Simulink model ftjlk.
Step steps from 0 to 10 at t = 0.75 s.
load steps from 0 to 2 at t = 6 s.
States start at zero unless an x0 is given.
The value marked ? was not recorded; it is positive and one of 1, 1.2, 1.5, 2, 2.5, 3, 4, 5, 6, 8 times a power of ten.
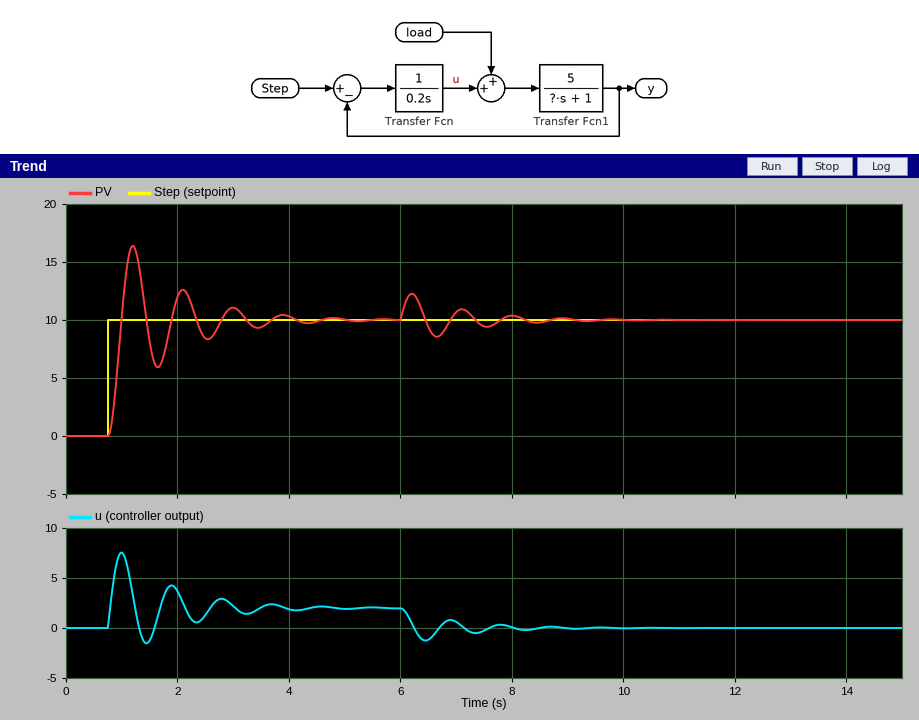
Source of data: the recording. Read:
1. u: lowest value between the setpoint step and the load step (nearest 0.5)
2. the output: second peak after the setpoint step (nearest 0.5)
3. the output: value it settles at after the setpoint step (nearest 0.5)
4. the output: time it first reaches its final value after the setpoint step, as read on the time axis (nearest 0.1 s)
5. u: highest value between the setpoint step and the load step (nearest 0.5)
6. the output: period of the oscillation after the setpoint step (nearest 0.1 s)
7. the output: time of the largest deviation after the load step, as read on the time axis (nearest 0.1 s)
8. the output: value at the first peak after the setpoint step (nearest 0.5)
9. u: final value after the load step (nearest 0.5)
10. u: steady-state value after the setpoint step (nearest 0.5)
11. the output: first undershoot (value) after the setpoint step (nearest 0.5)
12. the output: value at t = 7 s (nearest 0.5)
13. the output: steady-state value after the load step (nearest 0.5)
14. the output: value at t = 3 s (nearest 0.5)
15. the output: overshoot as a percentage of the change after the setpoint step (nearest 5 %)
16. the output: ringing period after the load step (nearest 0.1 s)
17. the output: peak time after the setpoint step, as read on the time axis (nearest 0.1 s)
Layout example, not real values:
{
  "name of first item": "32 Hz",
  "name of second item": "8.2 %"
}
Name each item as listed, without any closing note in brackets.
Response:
{
  "u: lowest value between the setpoint step and the load step": "-1.5",
  "the output: second peak after the setpoint step": "12.5",
  "the output: value it settles at after the setpoint step": "10.0",
  "the output: time it first reaches its final value after the setpoint step, as read on the time axis": "1.0 s",
  "u: highest value between the setpoint step and the load step": "7.5",
  "the output: period of the oscillation after the setpoint step": "0.9 s",
  "the output: time of the largest deviation after the load step, as read on the time axis": "6.2 s",
  "the output: value at the first peak after the setpoint step": "16.5",
  "u: final value after the load step": "0.0",
  "u: steady-state value after the setpoint step": "2.0",
  "the output: first undershoot (value) after the setpoint step": "6.0",
  "the output: value at t = 7 s": "10.5",
  "the output: steady-state value after the load step": "10.0",
  "the output: value at t = 3 s": "11.0",
  "the output: overshoot as a percentage of the change after the setpoint step": "65 %",
  "the output: ringing period after the load step": "0.9 s",
  "the output: peak time after the setpoint step, as read on the time axis": "1.2 s"
}
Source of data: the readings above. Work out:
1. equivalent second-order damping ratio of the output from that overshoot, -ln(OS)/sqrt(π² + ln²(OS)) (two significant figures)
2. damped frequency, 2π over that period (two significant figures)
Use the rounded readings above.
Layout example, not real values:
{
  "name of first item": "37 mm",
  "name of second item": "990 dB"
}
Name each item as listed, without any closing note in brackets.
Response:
{
  "equivalent second-order damping ratio of the output from that overshoot, -ln(OS)/sqrt(π² + ln²(OS))": "0.14",
  "damped frequency, 2π over that period": "7.0 rad/s"
}
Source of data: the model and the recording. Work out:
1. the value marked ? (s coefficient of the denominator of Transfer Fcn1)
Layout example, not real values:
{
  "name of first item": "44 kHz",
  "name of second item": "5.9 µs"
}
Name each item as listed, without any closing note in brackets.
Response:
{
  "the value marked ?": "0.5"
}
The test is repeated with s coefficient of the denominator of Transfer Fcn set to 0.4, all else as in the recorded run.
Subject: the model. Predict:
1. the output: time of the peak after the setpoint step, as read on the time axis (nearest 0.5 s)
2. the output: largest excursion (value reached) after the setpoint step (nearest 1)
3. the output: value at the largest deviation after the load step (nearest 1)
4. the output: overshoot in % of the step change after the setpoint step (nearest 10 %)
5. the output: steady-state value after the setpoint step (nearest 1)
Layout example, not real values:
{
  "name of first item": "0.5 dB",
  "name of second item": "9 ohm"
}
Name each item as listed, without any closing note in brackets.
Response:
{
  "the output: time of the peak after the setpoint step, as read on the time axis": "1.5 s",
  "the output: largest excursion (value reached) after the setpoint step": "15",
  "the output: value at the largest deviation after the load step": "13",
  "the output: overshoot in % of the step change after the setpoint step": "50 %",
  "the output: steady-state value after the setpoint step": "10"
}
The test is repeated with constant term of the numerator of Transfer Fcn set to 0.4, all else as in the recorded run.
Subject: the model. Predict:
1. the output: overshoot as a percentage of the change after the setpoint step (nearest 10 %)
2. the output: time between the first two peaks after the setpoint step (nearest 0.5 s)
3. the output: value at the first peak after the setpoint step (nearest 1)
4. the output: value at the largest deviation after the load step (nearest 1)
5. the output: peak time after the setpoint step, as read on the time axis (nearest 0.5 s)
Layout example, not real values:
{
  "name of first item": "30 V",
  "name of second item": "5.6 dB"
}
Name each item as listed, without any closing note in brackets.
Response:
{
  "the output: overshoot as a percentage of the change after the setpoint step": "50 %",
  "the output: time between the first two peaks after the setpoint step": "1.5 s",
  "the output: value at the first peak after the setpoint step": "15",
  "the output: value at the largest deviation after the load step": "13",
  "the output: peak time after the setpoint step, as read on the time axis": "1.5 s"
}
